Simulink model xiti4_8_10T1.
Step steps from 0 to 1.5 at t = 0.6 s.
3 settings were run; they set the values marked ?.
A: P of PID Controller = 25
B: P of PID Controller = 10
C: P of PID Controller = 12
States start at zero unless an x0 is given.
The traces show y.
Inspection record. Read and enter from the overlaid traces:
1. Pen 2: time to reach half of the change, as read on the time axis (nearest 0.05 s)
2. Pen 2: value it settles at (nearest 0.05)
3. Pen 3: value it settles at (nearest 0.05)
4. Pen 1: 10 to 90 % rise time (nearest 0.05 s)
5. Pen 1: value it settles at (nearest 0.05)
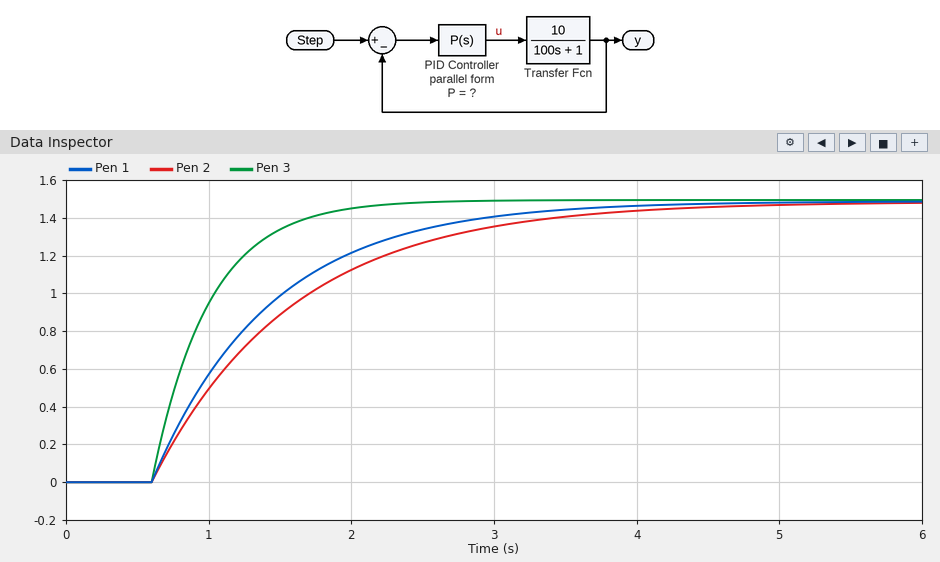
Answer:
1.30 s
1.50
1.50
1.80 s
1.50
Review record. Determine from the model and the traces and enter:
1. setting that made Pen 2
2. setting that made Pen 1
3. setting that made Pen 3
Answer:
B
C
A
